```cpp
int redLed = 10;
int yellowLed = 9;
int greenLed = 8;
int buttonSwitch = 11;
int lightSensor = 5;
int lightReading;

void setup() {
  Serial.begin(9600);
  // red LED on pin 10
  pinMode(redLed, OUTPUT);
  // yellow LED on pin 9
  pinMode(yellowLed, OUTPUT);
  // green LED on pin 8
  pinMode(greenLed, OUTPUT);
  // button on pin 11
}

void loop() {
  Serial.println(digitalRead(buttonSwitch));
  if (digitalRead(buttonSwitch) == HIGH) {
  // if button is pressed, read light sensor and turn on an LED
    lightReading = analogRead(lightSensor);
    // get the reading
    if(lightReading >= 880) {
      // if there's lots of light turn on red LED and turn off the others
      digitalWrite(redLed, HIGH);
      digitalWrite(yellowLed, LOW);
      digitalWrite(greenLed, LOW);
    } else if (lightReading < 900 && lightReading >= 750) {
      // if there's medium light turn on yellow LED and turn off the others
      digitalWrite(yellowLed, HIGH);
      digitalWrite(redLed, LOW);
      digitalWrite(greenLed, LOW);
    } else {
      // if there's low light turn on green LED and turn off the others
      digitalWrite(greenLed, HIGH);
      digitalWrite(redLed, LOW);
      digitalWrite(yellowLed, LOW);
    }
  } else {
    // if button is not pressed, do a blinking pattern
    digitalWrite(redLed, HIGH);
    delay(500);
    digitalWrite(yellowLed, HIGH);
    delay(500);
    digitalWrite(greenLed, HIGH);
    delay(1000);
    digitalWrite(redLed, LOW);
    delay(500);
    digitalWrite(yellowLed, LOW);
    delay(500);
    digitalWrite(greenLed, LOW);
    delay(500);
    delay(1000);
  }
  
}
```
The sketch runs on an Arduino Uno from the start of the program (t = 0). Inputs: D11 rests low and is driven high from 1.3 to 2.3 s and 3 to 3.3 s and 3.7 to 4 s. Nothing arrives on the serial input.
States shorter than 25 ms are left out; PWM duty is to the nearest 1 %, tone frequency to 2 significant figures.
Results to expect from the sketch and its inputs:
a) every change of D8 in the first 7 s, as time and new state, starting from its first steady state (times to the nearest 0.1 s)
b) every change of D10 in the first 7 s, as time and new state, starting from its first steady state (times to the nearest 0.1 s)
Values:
0 s low; 1 s high; 3 s low; 5.5 s high
0 s high; 2 s low; 4.5 s high; 6.5 s low
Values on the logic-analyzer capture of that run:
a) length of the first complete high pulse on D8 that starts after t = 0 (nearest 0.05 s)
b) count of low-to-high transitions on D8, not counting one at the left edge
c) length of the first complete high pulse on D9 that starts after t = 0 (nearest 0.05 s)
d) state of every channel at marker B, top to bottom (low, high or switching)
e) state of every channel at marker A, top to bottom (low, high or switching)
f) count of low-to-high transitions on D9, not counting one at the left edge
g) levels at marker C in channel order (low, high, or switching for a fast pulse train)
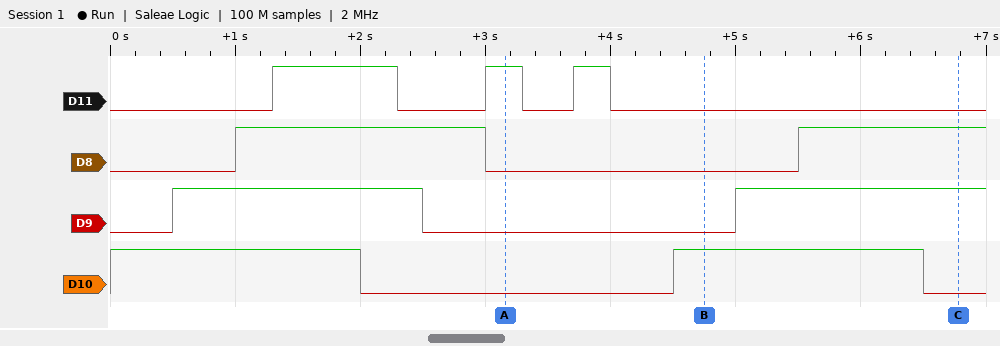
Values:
2.00 s
2
2.00 s
D11 low, D8 low, D9 low, D10 high
D11 high, D8 low, D9 low, D10 low
2
D11 low, D8 high, D9 high, D10 low
